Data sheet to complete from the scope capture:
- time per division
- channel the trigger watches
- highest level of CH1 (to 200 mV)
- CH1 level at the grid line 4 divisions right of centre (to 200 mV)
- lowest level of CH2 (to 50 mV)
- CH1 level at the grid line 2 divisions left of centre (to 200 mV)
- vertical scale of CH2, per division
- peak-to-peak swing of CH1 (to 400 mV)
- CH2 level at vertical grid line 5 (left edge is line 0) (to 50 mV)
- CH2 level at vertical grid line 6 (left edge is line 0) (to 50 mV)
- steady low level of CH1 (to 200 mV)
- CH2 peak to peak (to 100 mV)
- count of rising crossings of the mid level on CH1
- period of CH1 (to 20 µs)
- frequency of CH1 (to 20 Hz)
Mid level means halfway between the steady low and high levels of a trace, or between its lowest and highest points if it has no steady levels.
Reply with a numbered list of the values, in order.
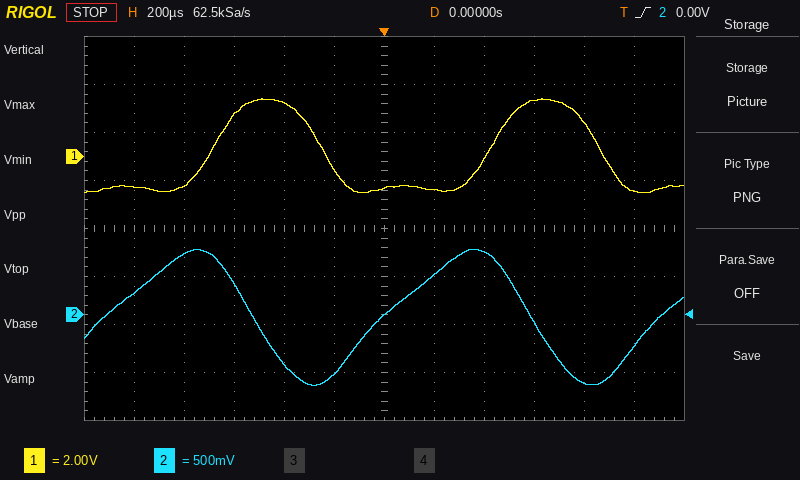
1. 200 µs
2. CH2
3. 2.4 V
4. 1.4 V
5. -750 mV
6. 2.2 V
7. 500 mV
8. 4.0 V
9. -600 mV
10. 0 mV
11. -1.4 V
12. 1.40 V
13. 2
14. 1.12 ms
15. 900 Hz
